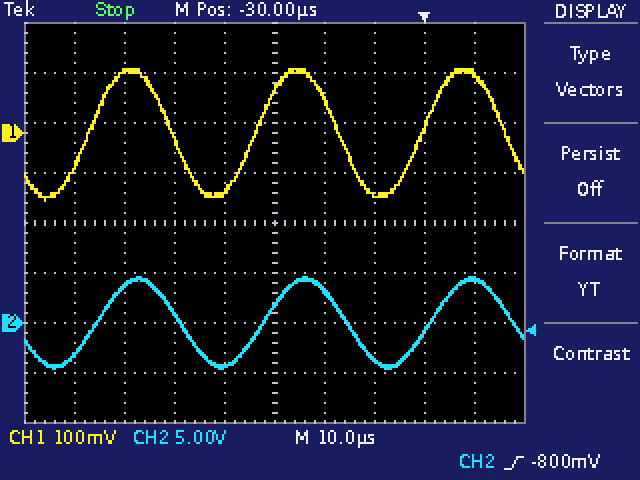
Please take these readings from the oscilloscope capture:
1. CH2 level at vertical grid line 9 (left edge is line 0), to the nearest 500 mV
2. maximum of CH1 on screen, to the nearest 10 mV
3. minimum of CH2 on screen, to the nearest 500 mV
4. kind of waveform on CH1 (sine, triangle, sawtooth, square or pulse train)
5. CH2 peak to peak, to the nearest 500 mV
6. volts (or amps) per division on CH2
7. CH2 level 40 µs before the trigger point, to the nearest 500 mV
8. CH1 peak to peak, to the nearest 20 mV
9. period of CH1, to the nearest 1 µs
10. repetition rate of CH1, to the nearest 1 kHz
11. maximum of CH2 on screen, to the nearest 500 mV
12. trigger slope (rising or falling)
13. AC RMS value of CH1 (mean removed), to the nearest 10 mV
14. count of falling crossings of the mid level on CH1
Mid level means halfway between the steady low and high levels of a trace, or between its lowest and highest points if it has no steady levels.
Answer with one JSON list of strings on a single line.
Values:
["4.5 V", "130 mV", "-4.5 V", "sine", "9.0 V", "5 V", "-4.5 V", "260 mV", "33 µs", "30 kHz", "4.5 V", "rising", "90 mV", "3"]
